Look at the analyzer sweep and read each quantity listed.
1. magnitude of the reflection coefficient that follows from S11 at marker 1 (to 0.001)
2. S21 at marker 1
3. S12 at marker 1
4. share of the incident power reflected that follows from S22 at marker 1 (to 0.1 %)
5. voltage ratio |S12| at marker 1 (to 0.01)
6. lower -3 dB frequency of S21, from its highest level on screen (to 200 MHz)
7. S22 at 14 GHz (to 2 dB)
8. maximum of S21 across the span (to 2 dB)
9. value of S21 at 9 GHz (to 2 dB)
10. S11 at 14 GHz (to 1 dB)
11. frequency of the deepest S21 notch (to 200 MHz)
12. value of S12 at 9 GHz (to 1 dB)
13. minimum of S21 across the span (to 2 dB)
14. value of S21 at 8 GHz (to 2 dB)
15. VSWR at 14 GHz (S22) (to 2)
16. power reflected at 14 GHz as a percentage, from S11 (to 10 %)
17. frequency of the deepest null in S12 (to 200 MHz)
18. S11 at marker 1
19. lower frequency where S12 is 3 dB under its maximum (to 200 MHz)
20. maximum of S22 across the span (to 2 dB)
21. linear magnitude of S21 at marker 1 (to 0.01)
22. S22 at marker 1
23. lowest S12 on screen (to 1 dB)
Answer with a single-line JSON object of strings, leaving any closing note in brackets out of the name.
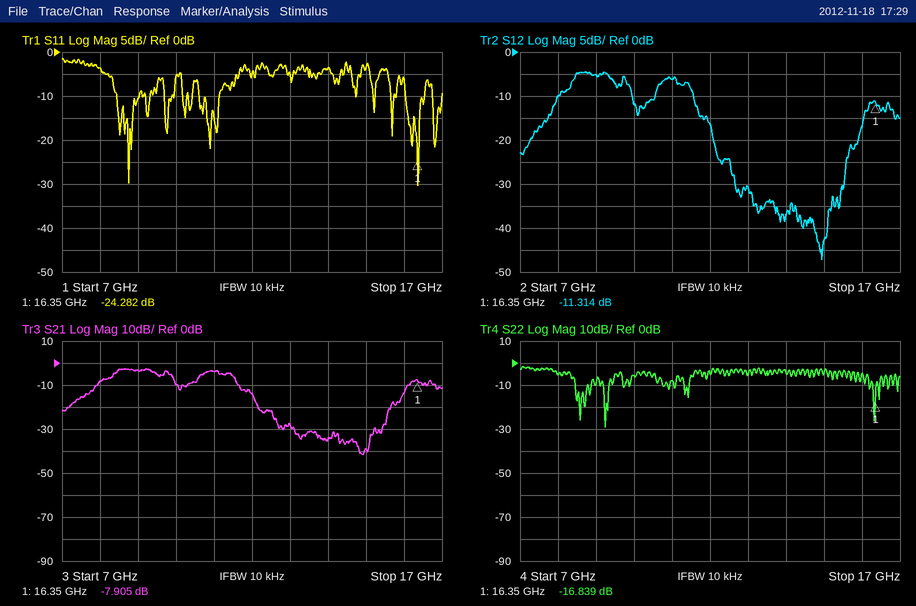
{"magnitude of the reflection coefficient that follows from S11 at marker 1": "0.061", "S21 at marker 1": "-7.905 dB", "S12 at marker 1": "-11.314 dB", "share of the incident power reflected that follows from S22 at marker 1": "2.1 %", "voltage ratio |S12| at marker 1": "0.27", "lower -3 dB frequency of S21, from its highest level on screen": "8.4 GHz", "S22 at 14 GHz": "-4 dB", "maximum of S21 across the span": "-2 dB", "value of S21 at 9 GHz": "-4 dB", "S11 at 14 GHz": "-4 dB", "frequency of the deepest S21 notch": "15.0 GHz", "value of S12 at 9 GHz": "-5 dB", "minimum of S21 across the span": "-42 dB", "value of S21 at 8 GHz": "-8 dB", "VSWR at 14 GHz (S22)": "4", "power reflected at 14 GHz as a percentage, from S11": "40 %", "frequency of the deepest null in S12": "15.0 GHz", "S11 at marker 1": "-24.282 dB", "lower frequency where S12 is 3 dB under its maximum": "8.4 GHz", "maximum of S22 across the span": "-2 dB", "linear magnitude of S21 at marker 1": "0.40", "S22 at marker 1": "-16.839 dB", "lowest S12 on screen": "-47 dB"}
